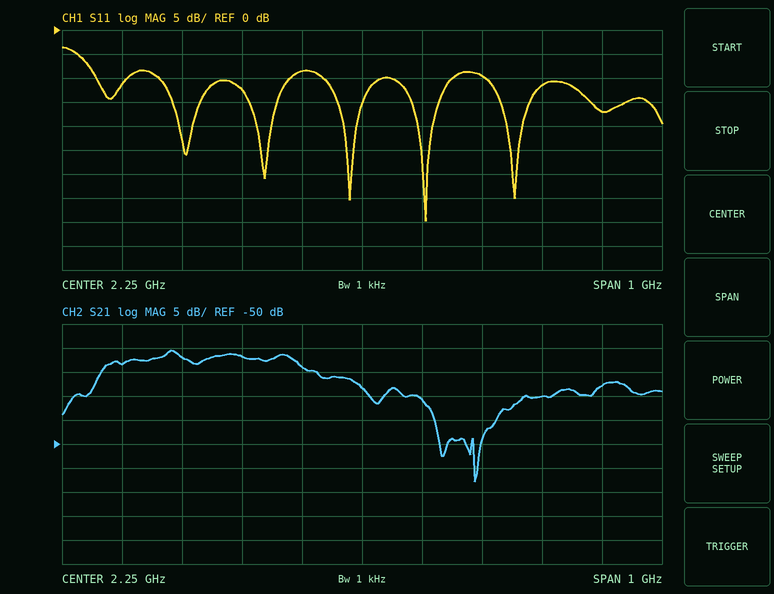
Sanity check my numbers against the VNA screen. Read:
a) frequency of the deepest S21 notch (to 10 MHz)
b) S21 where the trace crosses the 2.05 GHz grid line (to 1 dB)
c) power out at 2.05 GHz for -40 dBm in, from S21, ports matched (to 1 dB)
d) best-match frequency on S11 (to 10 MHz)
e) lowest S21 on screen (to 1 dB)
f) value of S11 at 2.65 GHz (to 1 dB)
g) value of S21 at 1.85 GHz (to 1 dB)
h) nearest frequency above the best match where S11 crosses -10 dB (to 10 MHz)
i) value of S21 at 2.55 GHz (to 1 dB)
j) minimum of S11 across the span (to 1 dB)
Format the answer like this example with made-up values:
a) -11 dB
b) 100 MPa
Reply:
a) 2.44 GHz
b) -32 dB
c) -72 dBm
d) 2.36 GHz
e) -58 dB
f) -17 dB
g) -33 dB
h) 2.40 GHz
i) -40 dB
j) -40 dB
